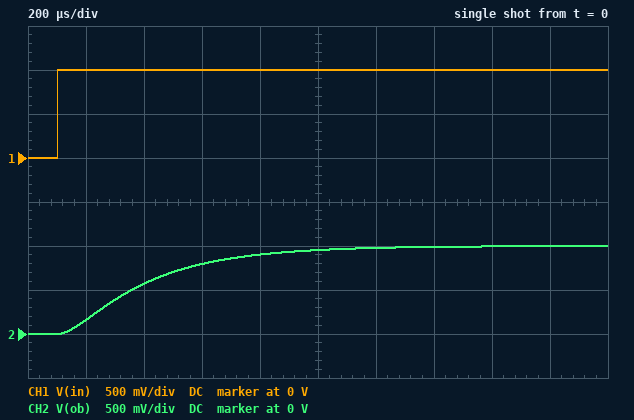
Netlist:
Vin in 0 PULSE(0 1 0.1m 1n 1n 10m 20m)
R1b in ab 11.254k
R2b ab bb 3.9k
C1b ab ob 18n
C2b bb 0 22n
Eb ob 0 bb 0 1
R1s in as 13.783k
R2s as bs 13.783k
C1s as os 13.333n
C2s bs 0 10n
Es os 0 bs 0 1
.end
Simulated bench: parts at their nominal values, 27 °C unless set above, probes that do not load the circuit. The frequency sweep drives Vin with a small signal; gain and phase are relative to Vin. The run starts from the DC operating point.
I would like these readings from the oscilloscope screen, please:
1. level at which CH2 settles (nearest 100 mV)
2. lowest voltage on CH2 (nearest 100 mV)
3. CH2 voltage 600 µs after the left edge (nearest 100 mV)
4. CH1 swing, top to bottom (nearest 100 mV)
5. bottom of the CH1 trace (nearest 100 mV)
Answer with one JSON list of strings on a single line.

["1.0 V", "0 V", "800 mV", "1.0 V", "0 V"]
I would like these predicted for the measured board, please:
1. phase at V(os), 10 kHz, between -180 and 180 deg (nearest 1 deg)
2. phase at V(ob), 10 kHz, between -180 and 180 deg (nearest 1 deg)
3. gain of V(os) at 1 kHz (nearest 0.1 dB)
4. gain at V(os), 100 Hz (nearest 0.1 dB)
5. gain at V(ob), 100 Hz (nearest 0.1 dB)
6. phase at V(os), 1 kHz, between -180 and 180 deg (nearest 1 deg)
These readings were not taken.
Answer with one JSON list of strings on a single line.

["-170 deg", "-163 deg", "-4.8 dB", "0 dB", "-0.1 dB", "-90 deg"]
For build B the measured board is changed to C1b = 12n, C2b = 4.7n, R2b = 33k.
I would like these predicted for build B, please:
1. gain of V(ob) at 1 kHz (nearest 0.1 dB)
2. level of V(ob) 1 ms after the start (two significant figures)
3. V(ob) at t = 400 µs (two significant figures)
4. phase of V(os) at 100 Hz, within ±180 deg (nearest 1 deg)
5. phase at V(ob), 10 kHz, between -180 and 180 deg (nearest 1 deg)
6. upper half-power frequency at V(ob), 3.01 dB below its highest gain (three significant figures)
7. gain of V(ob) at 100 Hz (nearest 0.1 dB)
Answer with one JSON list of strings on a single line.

["-2.4 dB", "1.0 V", "740 mV", "-10 deg", "-171 deg", "1.08 kHz", "0 dB"]
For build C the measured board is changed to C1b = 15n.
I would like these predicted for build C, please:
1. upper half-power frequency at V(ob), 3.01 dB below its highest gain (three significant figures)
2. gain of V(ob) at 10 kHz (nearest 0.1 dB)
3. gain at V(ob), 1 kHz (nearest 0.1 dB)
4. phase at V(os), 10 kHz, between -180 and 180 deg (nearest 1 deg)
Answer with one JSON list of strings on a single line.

["547 Hz", "-35.6 dB", "-6.6 dB", "-170 deg"]
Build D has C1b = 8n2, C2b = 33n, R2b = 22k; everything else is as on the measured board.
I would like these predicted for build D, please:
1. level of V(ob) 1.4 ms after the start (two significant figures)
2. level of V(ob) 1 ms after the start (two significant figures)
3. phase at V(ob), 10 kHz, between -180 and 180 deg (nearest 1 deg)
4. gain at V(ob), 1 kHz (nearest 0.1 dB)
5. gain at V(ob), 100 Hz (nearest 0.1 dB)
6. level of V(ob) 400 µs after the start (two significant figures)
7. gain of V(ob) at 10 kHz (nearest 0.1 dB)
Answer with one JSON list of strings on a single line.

["700 mV", "550 mV", "-165 deg", "-17.0 dB", "-1.5 dB", "200 mV", "-48.7 dB"]
